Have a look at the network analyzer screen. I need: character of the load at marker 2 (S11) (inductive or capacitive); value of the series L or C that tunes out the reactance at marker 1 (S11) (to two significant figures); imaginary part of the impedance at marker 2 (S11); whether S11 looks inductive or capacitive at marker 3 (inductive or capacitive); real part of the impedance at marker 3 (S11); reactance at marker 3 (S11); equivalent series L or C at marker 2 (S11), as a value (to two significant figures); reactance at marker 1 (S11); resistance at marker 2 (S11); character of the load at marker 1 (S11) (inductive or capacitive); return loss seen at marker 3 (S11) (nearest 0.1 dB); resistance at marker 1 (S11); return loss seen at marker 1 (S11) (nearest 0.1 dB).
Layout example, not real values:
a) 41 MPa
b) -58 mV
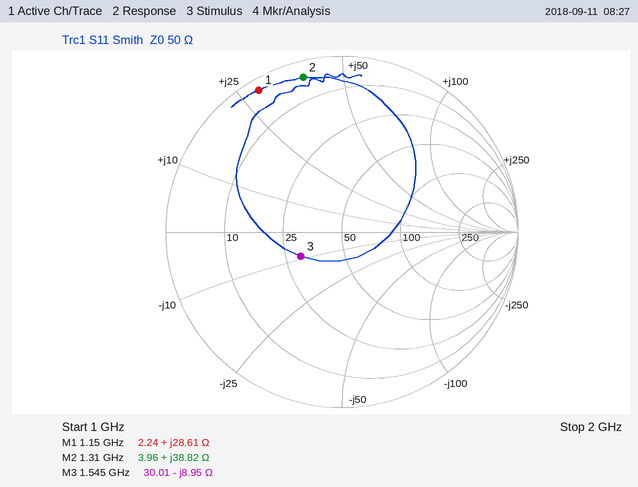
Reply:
a) inductive
b) 4.8 pF
c) +38.82 Ω
d) capacitive
e) 30.01 Ω
f) -8.95 Ω
g) 4.7 nH
h) +28.61 Ω
i) 3.96 Ω
j) inductive
k) 11.3 dB
l) 2.24 Ω
m) 0.6 dB
